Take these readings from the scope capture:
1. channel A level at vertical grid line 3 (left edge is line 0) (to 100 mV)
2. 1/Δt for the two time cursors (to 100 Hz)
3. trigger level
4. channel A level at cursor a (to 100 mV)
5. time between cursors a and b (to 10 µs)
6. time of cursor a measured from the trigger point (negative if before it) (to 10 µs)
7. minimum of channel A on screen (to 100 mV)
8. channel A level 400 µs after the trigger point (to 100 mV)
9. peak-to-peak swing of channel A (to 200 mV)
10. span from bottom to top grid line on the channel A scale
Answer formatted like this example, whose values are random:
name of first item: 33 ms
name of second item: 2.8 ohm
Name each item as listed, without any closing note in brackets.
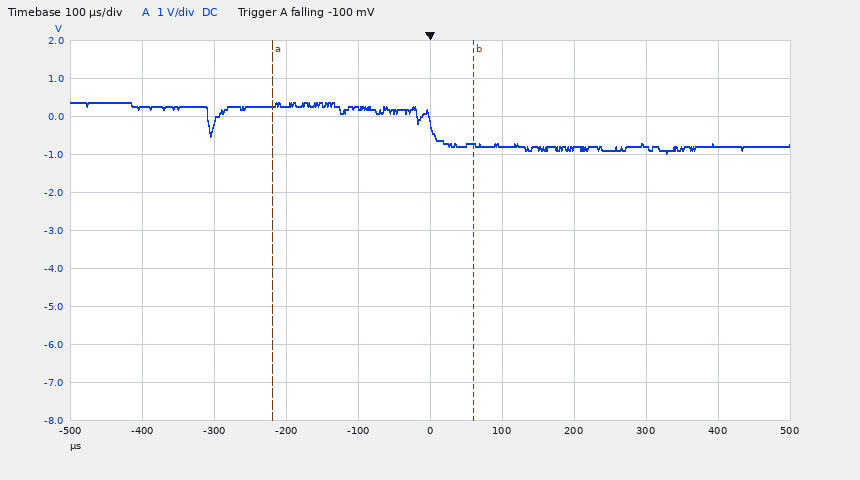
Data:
channel A level at vertical grid line 3 (left edge is line 0): 300 mV
1/Δt for the two time cursors: 3.6 kHz
trigger level: -100 mV
channel A level at cursor a: 300 mV
time between cursors a and b: 280 µs
time of cursor a measured from the trigger point (negative if before it): -220 µs
minimum of channel A on screen: -1.0 V
channel A level 400 µs after the trigger point: -800 mV
peak-to-peak swing of channel A: 1.4 V
span from bottom to top grid line on the channel A scale: 10 V
